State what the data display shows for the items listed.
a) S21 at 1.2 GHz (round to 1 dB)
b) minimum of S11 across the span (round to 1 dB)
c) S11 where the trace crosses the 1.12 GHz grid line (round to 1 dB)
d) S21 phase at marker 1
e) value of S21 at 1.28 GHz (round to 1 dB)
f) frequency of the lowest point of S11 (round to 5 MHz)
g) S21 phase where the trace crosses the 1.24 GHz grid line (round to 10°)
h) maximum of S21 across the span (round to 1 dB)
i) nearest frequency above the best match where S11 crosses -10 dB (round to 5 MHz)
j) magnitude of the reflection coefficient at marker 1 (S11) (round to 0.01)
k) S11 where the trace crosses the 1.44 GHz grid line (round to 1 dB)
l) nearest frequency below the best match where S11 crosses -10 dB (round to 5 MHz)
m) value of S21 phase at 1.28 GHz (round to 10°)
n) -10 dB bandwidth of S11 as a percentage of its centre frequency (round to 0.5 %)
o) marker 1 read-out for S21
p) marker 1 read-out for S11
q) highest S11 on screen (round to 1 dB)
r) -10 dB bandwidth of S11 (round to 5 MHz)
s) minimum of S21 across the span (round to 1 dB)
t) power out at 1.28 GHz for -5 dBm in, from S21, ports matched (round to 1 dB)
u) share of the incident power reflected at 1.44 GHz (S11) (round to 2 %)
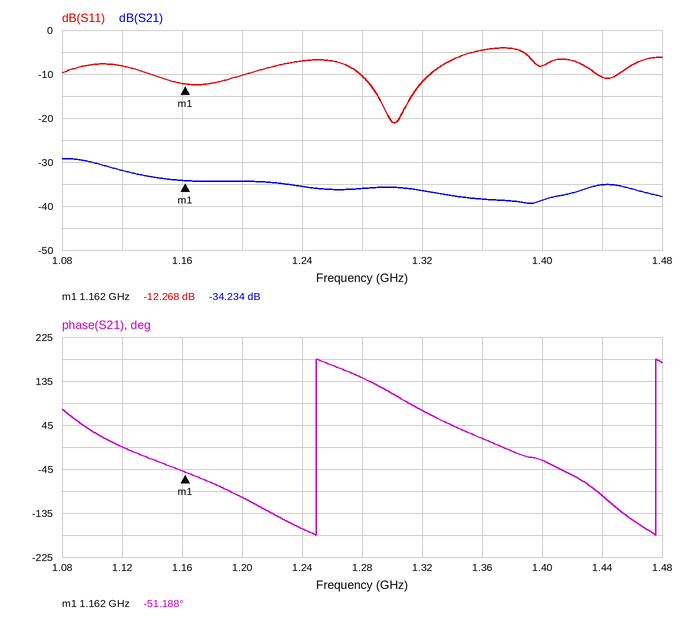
-34 dB
-21 dB
-8 dB
-51.188°
-36 dB
1.300 GHz
-170°
-29 dB
1.325 GHz
0.24
-11 dB
1.280 GHz
140°
3.5 %
-34.234 dB
-12.268 dB
-4 dB
45 MHz
-39 dB
-41 dBm
8 %
